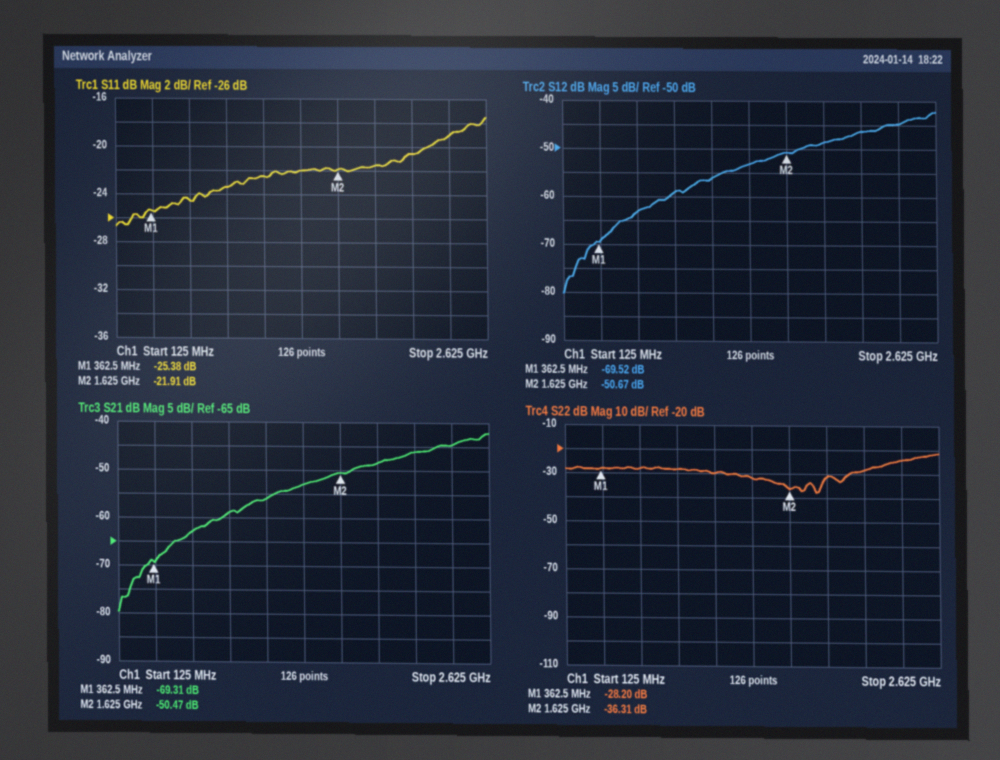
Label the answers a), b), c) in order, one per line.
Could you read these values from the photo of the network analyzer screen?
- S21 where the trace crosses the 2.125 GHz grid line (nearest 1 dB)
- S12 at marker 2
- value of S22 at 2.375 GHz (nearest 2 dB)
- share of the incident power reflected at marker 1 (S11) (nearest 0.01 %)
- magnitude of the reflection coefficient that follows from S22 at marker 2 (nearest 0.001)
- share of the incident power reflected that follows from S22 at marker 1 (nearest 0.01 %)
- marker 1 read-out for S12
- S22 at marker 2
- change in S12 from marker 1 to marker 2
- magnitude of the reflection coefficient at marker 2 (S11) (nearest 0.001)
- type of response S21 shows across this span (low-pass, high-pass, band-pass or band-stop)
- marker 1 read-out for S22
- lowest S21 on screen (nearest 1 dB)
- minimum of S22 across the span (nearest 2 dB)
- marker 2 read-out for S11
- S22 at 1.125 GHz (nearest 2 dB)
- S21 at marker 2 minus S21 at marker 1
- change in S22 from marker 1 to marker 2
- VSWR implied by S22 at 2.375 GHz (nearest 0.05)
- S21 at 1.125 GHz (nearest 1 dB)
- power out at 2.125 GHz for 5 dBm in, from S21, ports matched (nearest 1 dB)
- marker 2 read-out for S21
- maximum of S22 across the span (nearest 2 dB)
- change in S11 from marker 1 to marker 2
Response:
a) -46 dB
b) -50.67 dB
c) -24 dB
d) 0.29 %
e) 0.015
f) 0.15 %
g) -69.52 dB
h) -36.31 dB
i) 18.85 dB
j) 0.080
k) high-pass
l) -28.20 dB
m) -80 dB
n) -38 dB
o) -21.91 dB
p) -30 dB
q) 18.84 dB
r) -8.11 dB
s) 1.15
t) -56 dB
u) -41 dBm
v) -50.47 dB
w) -22 dB
x) 3.47 dB
